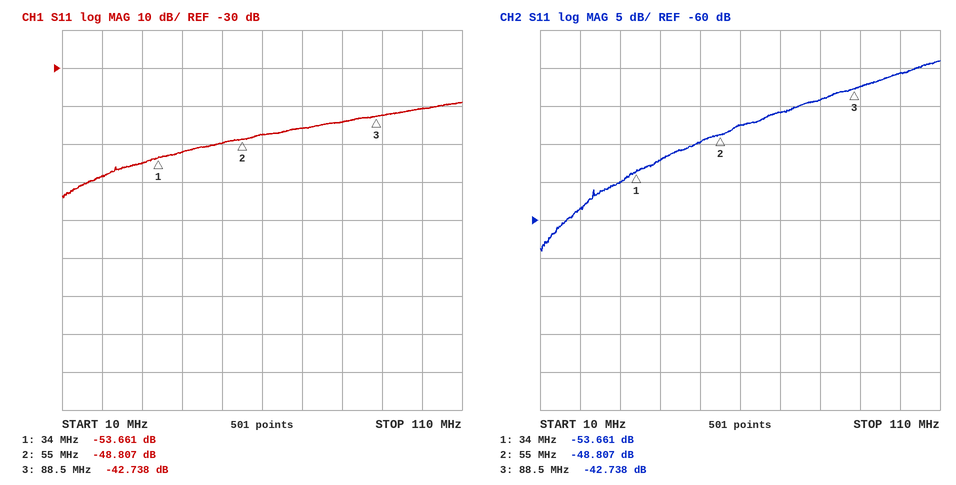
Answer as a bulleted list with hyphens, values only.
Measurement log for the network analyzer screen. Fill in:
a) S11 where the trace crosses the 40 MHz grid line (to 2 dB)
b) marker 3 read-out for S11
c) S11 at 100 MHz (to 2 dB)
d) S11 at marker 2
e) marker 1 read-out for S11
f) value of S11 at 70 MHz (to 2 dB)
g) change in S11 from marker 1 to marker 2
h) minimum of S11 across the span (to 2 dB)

- -52 dB
- -42.738 dB
- -40 dB
- -48.807 dB
- -53.661 dB
- -46 dB
- 4.854 dB
- -64 dB
